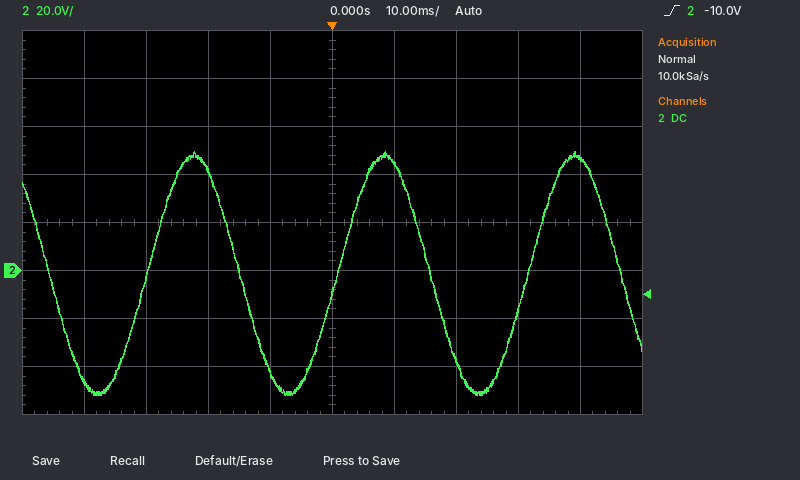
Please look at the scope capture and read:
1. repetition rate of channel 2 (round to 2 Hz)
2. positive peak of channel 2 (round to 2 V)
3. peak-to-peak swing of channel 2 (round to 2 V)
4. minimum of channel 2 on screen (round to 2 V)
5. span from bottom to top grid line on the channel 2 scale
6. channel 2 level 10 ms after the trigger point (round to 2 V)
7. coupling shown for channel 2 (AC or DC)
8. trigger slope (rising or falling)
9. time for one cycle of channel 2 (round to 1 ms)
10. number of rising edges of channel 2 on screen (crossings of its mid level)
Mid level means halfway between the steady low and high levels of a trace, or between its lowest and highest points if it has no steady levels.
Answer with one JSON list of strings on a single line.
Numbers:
["32 Hz", "50 V", "102 V", "-52 V", "160 V", "44 V", "DC", "rising", "31 ms", "3"]
